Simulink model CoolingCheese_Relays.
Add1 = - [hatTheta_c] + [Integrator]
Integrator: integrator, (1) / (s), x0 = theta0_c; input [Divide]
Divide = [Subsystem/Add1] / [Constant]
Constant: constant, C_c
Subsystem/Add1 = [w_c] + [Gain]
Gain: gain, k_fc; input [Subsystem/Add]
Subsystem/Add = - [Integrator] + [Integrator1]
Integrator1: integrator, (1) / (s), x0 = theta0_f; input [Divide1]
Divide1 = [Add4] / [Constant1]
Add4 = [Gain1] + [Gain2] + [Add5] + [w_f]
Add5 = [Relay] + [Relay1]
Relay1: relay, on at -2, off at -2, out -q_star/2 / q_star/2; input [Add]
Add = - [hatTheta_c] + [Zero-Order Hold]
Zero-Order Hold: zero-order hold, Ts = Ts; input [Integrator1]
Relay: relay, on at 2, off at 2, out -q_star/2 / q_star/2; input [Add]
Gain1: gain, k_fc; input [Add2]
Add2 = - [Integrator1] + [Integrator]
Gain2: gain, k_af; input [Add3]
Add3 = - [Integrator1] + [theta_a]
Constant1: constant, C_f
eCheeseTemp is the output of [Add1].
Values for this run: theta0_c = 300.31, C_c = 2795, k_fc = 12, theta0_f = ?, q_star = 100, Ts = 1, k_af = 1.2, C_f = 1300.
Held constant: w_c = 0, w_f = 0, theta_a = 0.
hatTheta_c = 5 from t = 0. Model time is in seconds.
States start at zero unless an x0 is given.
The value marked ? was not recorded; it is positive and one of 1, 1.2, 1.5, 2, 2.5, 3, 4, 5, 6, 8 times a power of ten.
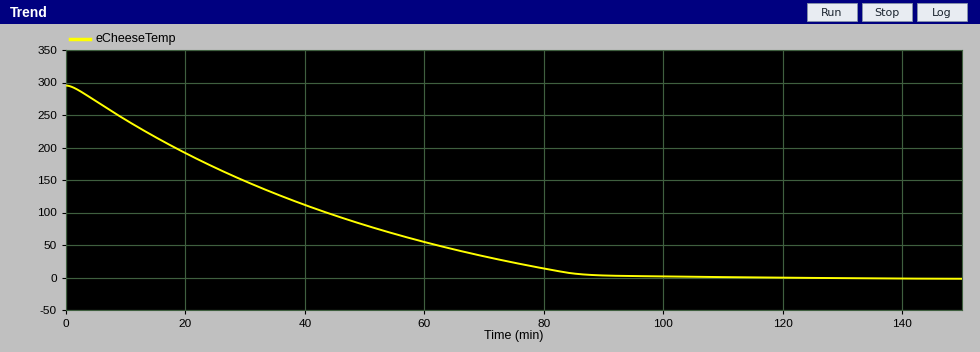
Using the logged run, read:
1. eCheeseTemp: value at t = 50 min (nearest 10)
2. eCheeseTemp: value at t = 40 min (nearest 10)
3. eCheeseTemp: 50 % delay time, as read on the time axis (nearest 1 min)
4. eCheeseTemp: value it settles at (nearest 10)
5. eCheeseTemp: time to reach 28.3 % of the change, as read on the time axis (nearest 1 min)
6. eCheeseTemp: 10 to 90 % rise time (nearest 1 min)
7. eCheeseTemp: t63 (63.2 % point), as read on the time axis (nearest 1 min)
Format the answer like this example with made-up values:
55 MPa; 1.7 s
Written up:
80; 110; 30 min; 0; 16 min; 66 min; 41 min
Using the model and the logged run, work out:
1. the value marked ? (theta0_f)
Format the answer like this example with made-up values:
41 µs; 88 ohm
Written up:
300
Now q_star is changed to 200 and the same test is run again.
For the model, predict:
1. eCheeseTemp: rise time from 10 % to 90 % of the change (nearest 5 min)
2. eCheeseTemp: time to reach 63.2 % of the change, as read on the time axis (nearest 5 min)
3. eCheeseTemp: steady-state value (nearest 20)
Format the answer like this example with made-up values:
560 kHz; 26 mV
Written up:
45 min; 30 min; 0
